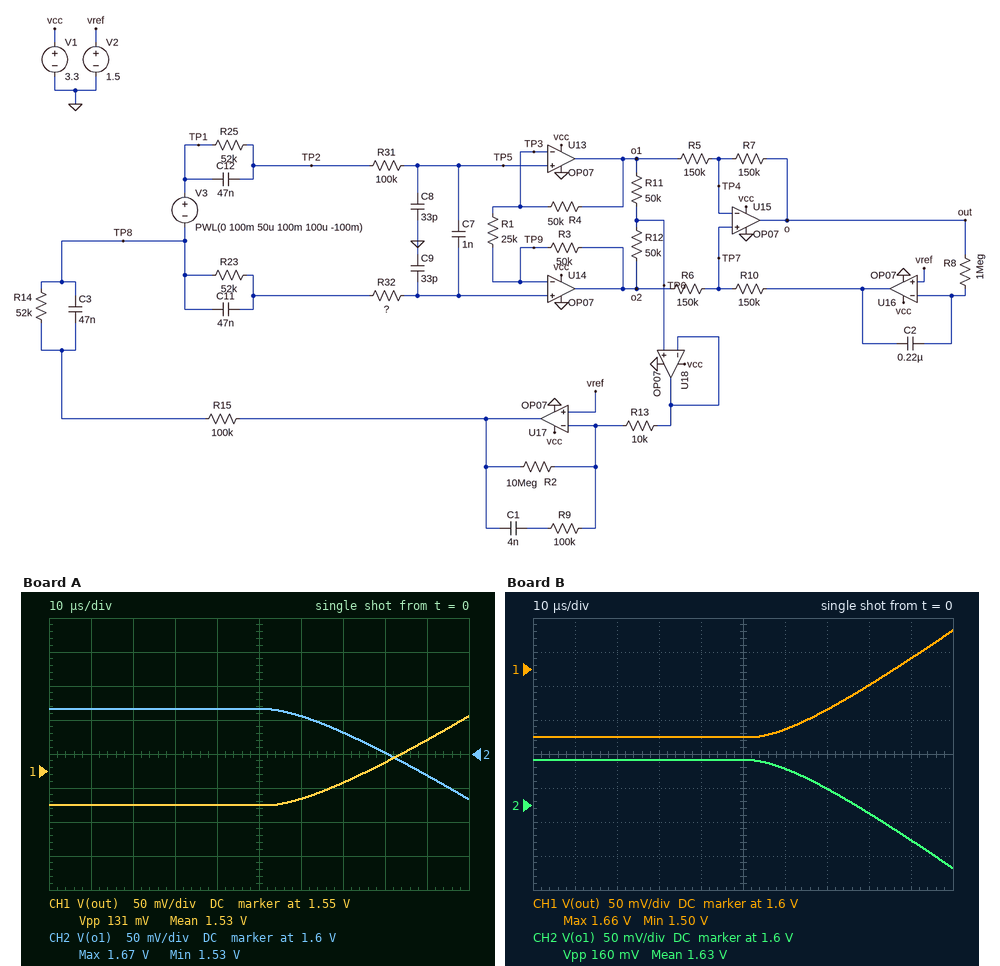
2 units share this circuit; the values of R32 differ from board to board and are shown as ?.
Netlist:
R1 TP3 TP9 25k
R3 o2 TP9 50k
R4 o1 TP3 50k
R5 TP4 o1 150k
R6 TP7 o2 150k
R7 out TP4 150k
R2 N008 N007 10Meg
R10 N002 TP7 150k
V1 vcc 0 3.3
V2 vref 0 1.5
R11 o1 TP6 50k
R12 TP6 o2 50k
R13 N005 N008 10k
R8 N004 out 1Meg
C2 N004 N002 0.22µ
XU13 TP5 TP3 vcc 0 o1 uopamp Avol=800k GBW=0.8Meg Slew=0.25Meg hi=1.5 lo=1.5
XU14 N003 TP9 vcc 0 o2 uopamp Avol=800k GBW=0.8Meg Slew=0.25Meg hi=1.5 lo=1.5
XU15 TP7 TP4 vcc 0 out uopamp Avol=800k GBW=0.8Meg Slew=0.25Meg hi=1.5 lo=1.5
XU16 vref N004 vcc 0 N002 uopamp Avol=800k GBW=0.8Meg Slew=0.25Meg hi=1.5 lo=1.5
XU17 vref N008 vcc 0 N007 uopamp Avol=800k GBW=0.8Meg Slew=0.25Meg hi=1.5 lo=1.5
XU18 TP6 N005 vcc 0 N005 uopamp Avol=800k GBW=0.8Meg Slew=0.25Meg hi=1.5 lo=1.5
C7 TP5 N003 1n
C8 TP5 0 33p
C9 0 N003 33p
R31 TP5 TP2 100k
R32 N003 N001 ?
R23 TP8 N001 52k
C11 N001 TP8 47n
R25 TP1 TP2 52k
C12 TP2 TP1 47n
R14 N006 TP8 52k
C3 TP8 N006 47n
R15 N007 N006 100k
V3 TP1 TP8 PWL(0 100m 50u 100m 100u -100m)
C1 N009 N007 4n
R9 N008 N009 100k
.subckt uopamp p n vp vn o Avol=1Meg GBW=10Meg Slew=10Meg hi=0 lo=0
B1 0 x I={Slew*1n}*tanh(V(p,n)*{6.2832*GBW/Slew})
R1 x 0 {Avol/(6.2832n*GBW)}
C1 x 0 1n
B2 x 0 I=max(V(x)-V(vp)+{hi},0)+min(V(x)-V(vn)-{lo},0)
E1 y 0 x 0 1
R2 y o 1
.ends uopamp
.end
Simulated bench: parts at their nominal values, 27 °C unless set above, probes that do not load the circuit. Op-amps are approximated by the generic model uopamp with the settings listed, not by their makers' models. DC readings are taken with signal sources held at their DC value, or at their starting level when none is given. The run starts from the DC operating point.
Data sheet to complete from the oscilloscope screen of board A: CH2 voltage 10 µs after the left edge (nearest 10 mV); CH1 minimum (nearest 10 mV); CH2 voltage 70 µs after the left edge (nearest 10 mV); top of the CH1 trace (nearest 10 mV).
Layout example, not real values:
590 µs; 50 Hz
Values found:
1.67 V; 1.50 V; 1.63 V; 1.63 V
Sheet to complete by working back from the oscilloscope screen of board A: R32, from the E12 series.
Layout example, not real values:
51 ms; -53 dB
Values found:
68 kΩ
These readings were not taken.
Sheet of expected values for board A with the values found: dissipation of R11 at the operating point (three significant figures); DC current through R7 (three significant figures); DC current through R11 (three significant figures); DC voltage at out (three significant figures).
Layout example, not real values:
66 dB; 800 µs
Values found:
139 nW; 555 nA; 1.67 µA; 1.50 V
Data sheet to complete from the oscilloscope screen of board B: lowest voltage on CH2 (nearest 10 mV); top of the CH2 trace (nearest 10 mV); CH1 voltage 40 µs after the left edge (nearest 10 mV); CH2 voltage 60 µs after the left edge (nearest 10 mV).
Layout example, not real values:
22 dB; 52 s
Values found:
1.51 V; 1.67 V; 1.50 V; 1.65 V
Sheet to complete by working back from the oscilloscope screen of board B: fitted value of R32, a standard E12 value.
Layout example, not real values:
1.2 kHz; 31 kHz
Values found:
120 kΩ
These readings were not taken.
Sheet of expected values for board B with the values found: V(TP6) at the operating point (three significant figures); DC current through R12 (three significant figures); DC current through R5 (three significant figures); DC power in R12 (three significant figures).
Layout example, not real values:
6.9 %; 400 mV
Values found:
1.58 V; 1.67 µA; 555 nA; 139 nW
